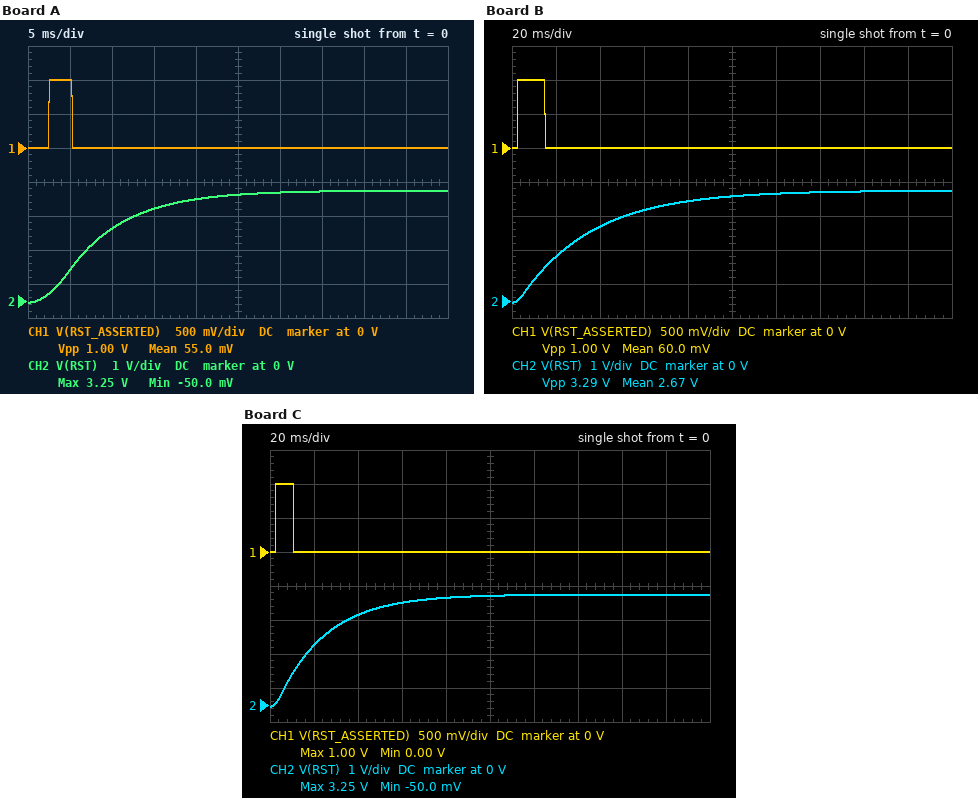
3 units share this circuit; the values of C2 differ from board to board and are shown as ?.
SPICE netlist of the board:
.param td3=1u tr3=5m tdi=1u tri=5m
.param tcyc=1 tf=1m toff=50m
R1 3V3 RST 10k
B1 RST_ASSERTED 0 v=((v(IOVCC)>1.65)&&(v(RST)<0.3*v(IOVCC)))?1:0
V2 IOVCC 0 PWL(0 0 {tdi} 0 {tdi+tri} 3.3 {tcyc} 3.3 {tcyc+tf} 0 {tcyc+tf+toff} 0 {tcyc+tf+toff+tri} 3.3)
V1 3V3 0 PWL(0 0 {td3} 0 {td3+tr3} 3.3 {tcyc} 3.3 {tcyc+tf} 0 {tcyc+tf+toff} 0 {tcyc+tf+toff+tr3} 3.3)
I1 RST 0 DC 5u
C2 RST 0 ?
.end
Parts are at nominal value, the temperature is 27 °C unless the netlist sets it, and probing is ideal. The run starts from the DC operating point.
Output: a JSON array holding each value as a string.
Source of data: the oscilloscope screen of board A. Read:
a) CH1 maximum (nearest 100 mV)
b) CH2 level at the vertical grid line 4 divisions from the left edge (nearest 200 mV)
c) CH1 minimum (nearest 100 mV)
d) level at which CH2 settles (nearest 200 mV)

["1.0 V", "3.0 V", "0 V", "3.2 V"]
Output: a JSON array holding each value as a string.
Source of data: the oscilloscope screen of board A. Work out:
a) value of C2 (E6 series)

["680 nF"]
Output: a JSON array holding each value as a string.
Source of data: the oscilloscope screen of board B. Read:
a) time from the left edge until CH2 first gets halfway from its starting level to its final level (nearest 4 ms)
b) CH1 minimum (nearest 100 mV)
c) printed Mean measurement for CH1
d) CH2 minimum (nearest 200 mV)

["24 ms", "0 V", "60.0 mV", "0 V"]
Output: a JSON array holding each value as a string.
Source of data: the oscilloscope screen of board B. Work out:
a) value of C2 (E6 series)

["3.3 µF"]
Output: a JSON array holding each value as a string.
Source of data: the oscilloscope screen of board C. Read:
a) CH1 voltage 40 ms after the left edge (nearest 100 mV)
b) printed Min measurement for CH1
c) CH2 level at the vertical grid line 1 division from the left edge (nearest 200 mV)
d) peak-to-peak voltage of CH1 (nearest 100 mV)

["0 V", "0.00 V", "1.8 V", "1.0 V"]
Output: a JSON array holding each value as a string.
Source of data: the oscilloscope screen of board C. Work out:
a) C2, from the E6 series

["2.2 µF"]
